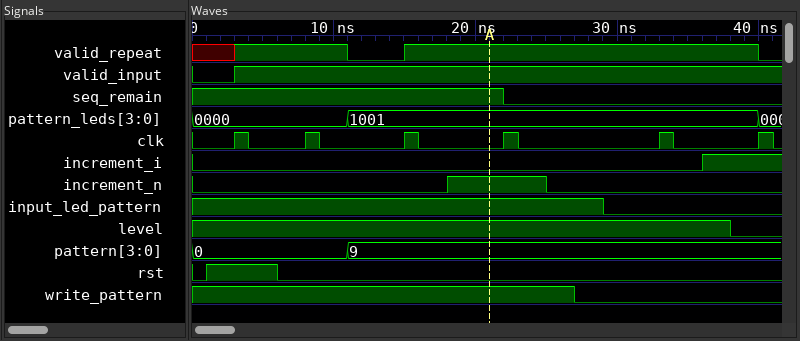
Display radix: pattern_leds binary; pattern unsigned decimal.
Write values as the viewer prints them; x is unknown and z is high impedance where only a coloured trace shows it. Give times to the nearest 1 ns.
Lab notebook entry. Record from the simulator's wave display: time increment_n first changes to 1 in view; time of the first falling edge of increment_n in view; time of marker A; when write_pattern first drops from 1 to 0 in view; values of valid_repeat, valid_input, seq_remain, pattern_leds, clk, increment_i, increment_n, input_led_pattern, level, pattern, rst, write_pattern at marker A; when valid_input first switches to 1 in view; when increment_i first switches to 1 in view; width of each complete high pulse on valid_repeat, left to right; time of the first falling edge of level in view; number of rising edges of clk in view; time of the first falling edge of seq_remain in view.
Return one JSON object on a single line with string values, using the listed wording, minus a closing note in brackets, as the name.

{"time increment_n first changes to 1 in view": "18 ns", "time of the first falling edge of increment_n in view": "25 ns", "time of marker A": "21 ns", "when write_pattern first drops from 1 to 0 in view": "27 ns", "values of valid_repeat, valid_input, seq_remain, pattern_leds, clk, increment_i, increment_n, input_led_pattern, level, pattern, rst, write_pattern at marker A": "valid_repeat=1, valid_input=1, seq_remain=1, pattern_leds=1001, clk=0, increment_i=0, increment_n=1, input_led_pattern=1, level=1, pattern=9, rst=0, write_pattern=1", "when valid_input first switches to 1 in view": "3 ns", "when increment_i first switches to 1 in view": "36 ns", "width of each complete high pulse on valid_repeat, left to right": "25 ns", "time of the first falling edge of level in view": "38 ns", "number of rising edges of clk in view": "6", "time of the first falling edge of seq_remain in view": "22 ns"}
